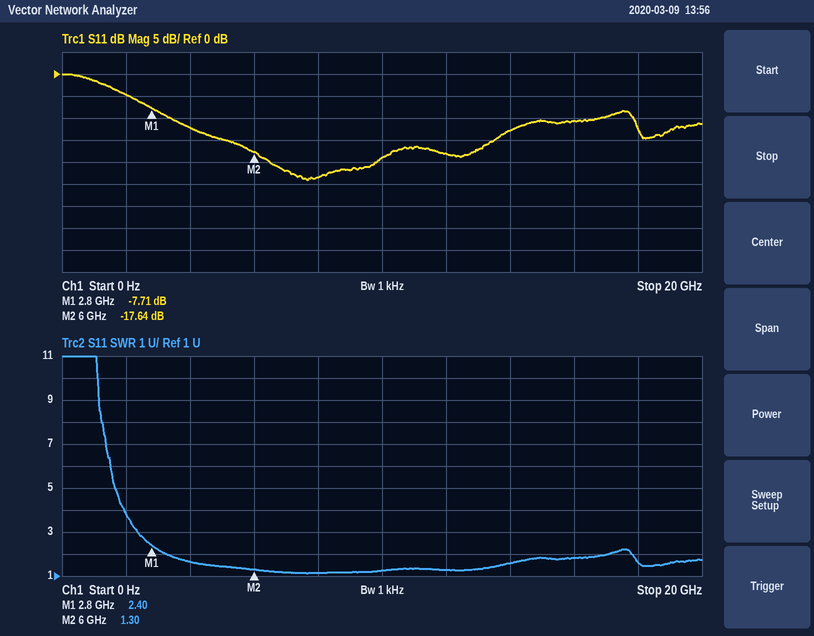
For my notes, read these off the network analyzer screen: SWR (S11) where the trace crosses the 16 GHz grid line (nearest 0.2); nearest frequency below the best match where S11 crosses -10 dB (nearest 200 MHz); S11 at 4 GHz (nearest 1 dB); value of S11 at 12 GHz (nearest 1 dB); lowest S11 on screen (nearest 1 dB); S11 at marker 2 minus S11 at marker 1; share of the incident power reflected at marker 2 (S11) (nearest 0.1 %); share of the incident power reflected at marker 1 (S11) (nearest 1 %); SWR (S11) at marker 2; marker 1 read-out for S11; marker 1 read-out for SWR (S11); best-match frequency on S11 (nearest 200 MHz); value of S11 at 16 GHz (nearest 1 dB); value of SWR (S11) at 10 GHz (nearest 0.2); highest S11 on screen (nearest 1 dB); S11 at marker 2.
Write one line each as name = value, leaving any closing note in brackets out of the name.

SWR (S11) where the trace crosses the 16 GHz grid line = 1.8
nearest frequency below the best match where S11 crosses -10 dB = 3.4 GHz
S11 at 4 GHz = -12 dB
value of S11 at 12 GHz = -18 dB
lowest S11 on screen = -24 dB
S11 at marker 2 minus S11 at marker 1 = -9.93 dB
share of the incident power reflected at marker 2 (S11) = 1.7 %
share of the incident power reflected at marker 1 (S11) = 17 %
SWR (S11) at marker 2 = 1.30
marker 1 read-out for S11 = -7.71 dB
marker 1 read-out for SWR = 2.40
best-match frequency on S11 = 7.6 GHz
value of S11 at 16 GHz = -11 dB
value of SWR (S11) at 10 GHz = 1.2
highest S11 on screen = 0 dB
S11 at marker 2 = -17.64 dB
